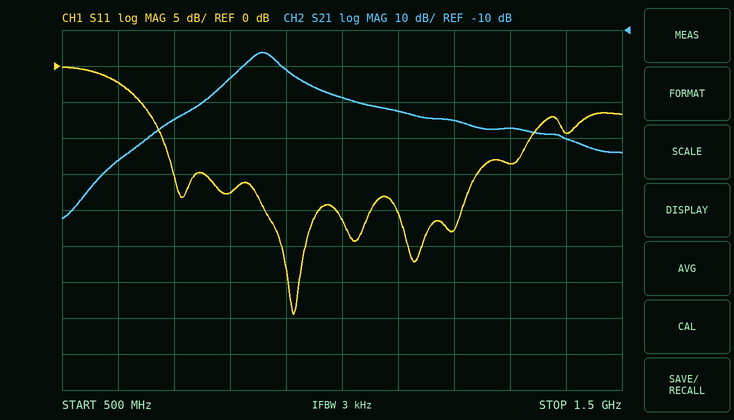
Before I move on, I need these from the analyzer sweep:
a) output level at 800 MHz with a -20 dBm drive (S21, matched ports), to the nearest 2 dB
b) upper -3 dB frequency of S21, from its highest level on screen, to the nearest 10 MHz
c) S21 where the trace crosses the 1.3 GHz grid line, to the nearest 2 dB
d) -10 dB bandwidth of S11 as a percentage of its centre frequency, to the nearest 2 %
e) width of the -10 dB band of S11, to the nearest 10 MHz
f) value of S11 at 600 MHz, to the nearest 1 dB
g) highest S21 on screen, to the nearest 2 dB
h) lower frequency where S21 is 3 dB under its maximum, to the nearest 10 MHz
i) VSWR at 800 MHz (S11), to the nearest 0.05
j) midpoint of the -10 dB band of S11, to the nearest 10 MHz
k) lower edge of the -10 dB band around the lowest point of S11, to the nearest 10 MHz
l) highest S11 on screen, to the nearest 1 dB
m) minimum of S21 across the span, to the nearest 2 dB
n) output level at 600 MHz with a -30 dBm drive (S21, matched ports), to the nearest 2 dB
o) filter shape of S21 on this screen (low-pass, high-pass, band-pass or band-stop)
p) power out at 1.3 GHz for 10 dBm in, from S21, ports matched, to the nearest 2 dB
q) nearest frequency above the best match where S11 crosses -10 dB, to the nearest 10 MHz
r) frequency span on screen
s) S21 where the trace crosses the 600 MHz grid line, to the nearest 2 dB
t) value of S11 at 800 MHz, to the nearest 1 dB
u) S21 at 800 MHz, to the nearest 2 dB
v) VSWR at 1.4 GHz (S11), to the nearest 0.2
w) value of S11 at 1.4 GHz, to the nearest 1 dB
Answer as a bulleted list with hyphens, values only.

- -44 dBm
- 890 MHz
- -38 dB
- 66 %
- 660 MHz
- -2 dB
- -16 dB
- 830 MHz
- 1.30
- 1.01 GHz
- 680 MHz
- 0 dB
- -62 dB
- -76 dBm
- band-pass
- -28 dBm
- 1.34 GHz
- 1 GHz
- -46 dB
- -18 dB
- -24 dB
- 2.0
- -9 dB
